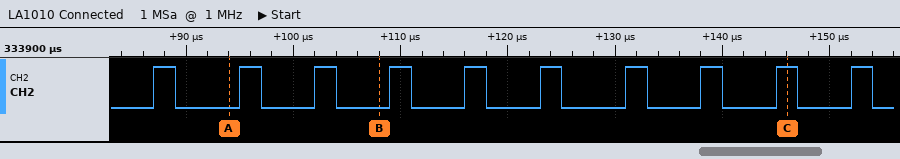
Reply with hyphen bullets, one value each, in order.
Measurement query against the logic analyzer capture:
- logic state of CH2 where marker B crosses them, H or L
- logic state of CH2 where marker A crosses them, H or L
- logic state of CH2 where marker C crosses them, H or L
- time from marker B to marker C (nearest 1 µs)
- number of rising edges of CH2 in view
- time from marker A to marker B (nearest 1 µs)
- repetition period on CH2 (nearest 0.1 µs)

- CH2=L
- CH2=L
- CH2=H
- 38 µs
- 10
- 14 µs
- 7.2 µs
